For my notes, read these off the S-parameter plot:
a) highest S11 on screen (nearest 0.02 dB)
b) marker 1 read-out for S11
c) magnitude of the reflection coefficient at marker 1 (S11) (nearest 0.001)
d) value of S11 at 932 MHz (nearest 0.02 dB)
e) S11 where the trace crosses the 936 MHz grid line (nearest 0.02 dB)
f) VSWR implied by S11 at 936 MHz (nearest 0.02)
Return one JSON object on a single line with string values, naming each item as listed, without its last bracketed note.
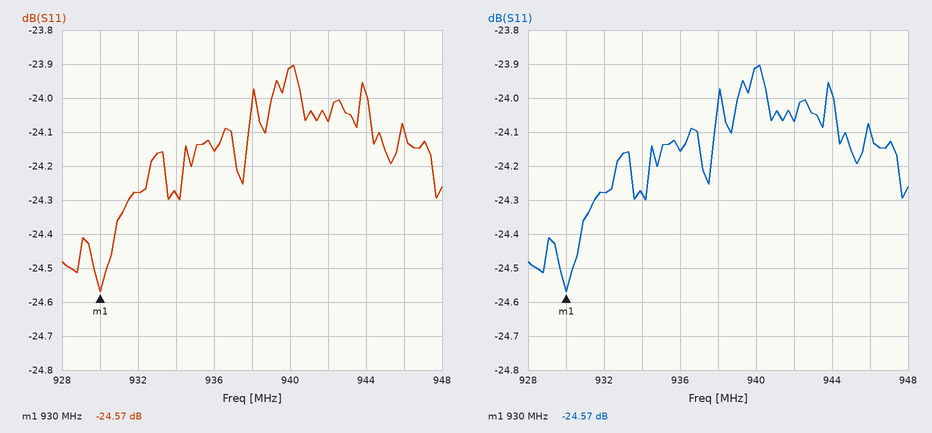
{"highest S11 on screen": "-23.90 dB", "marker 1 read-out for S11": "-24.57 dB", "magnitude of the reflection coefficient at marker 1 (S11)": "0.059", "value of S11 at 932 MHz": "-24.28 dB", "S11 where the trace crosses the 936 MHz grid line": "-24.16 dB", "VSWR implied by S11 at 936 MHz": "1.14"}
